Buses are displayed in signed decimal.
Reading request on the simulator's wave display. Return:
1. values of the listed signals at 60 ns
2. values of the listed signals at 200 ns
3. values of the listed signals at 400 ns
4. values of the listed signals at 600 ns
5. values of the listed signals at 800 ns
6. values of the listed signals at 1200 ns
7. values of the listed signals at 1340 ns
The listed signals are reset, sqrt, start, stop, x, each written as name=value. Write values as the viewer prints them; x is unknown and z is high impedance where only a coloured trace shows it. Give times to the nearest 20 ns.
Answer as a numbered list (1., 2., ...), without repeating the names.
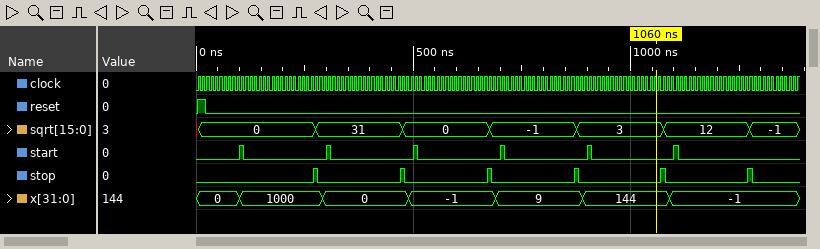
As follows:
1. reset=0, sqrt=0, start=0, stop=0, x=0
2. reset=0, sqrt=0, start=0, stop=0, x=1000
3. reset=0, sqrt=31, start=0, stop=0, x=0
4. reset=0, sqrt=0, start=0, stop=0, x=-1
5. reset=0, sqrt=-1, start=0, stop=0, x=9
6. reset=0, sqrt=12, start=0, stop=0, x=-1
7. reset=0, sqrt=-1, start=0, stop=0, x=-1
